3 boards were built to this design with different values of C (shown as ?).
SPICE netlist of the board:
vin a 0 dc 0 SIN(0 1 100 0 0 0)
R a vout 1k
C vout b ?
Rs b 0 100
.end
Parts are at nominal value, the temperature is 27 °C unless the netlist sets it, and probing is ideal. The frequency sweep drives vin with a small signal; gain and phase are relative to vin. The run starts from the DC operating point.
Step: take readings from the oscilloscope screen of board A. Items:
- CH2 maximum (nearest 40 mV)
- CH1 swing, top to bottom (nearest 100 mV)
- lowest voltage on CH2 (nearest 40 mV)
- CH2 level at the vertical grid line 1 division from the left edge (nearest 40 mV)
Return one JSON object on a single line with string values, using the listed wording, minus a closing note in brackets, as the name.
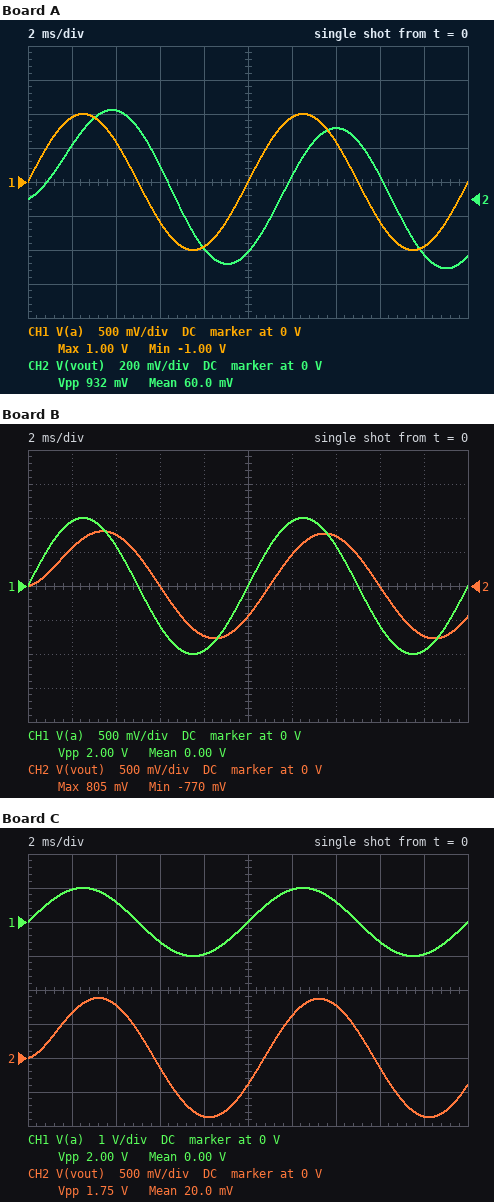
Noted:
{"CH2 maximum": "520 mV", "CH1 swing, top to bottom": "2.0 V", "lowest voltage on CH2": "-400 mV", "CH2 level at the vertical grid line 1 division from the left edge": "320 mV"}
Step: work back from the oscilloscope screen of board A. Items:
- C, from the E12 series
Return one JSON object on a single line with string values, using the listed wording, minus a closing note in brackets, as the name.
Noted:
{"C, from the E12 series": "3.3 µF"}
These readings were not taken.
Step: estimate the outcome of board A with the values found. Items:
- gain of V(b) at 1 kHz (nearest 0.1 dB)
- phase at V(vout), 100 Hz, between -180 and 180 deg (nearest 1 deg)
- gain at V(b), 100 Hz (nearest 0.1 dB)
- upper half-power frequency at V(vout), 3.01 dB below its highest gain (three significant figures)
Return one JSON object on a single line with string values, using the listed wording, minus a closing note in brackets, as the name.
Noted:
{"gain of V(b) at 1 kHz": "-20.8 dB", "phase at V(vout), 100 Hz, between -180 and 180 deg": "-55 deg", "gain at V(b), 100 Hz": "-21.6 dB", "upper half-power frequency at V(vout), 3.01 dB below its highest gain": "44.2 Hz"}
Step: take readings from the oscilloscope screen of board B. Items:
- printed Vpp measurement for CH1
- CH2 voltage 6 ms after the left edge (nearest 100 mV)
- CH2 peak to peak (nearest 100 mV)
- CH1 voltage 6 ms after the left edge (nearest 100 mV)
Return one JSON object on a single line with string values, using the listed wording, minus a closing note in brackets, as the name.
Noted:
{"printed Vpp measurement for CH1": "2.00 V", "CH2 voltage 6 ms after the left edge": "0 V", "CH2 peak to peak": "1.6 V", "CH1 voltage 6 ms after the left edge": "-600 mV"}
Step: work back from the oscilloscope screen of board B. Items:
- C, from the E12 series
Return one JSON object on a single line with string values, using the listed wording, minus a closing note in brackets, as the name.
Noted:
{"C, from the E12 series": "1.2 µF"}
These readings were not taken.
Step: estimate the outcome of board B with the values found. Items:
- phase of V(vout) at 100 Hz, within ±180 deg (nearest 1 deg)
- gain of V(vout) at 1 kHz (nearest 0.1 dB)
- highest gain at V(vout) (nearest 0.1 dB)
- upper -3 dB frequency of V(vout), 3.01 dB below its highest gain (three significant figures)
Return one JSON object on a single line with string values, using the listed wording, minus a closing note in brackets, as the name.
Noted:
{"phase of V(vout) at 100 Hz, within ±180 deg": "-35 deg", "gain of V(vout) at 1 kHz": "-16.5 dB", "highest gain at V(vout)": "0 dB", "upper -3 dB frequency of V(vout), 3.01 dB below its highest gain": "122 Hz"}
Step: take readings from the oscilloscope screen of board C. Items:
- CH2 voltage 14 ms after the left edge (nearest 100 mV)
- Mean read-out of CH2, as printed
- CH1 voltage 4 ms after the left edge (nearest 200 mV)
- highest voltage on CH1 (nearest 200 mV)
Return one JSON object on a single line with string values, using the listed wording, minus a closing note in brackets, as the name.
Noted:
{"CH2 voltage 14 ms after the left edge": "800 mV", "Mean read-out of CH2, as printed": "20.0 mV", "CH1 voltage 4 ms after the left edge": "600 mV", "highest voltage on CH1": "1.0 V"}
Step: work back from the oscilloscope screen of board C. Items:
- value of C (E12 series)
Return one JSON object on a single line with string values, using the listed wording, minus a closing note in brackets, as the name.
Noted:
{"value of C": "820 nF"}
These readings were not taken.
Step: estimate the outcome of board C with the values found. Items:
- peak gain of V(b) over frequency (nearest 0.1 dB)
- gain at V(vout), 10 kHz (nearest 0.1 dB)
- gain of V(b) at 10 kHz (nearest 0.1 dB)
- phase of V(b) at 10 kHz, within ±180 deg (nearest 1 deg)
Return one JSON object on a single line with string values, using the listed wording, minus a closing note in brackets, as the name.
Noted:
{"peak gain of V(b) over frequency": "-20.8 dB", "gain at V(vout), 10 kHz": "-20.7 dB", "gain of V(b) at 10 kHz": "-20.8 dB", "phase of V(b) at 10 kHz, within ±180 deg": "1 deg"}
